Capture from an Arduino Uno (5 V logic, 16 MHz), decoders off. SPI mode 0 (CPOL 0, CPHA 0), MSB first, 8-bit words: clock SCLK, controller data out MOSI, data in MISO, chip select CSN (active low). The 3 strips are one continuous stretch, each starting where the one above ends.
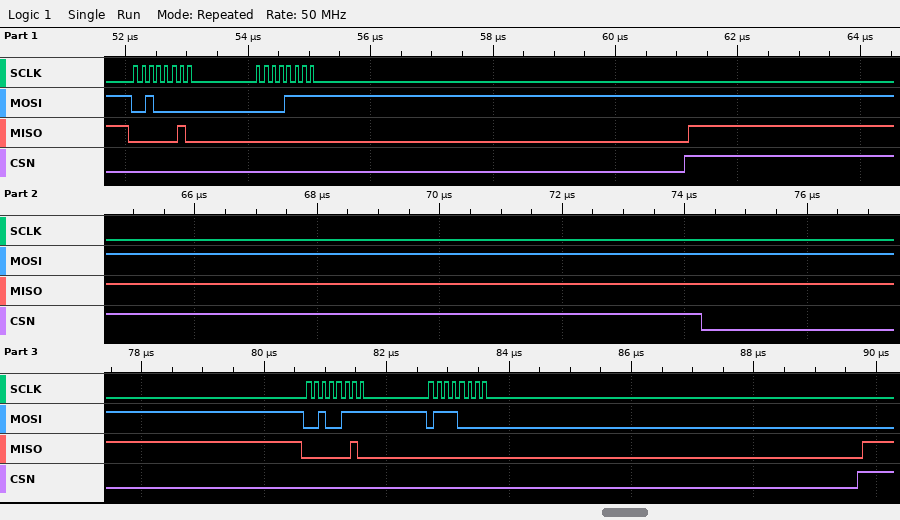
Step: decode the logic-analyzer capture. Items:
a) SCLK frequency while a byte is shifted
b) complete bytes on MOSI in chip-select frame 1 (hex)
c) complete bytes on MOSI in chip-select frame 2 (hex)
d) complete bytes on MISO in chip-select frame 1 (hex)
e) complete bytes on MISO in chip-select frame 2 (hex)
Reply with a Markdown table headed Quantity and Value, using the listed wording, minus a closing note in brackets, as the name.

| Quantity | Value |
|---|---|
| SCLK frequency while a byte is shifted | 8 MHz |
| complete bytes on MOSI in chip-select frame 1 | 0x20 0x0F |
| complete bytes on MOSI in chip-select frame 2 | 0x27 0x70 |
| complete bytes on MISO in chip-select frame 1 | 0x02 0x00 |
| complete bytes on MISO in chip-select frame 2 | 0x02 0x00 |
